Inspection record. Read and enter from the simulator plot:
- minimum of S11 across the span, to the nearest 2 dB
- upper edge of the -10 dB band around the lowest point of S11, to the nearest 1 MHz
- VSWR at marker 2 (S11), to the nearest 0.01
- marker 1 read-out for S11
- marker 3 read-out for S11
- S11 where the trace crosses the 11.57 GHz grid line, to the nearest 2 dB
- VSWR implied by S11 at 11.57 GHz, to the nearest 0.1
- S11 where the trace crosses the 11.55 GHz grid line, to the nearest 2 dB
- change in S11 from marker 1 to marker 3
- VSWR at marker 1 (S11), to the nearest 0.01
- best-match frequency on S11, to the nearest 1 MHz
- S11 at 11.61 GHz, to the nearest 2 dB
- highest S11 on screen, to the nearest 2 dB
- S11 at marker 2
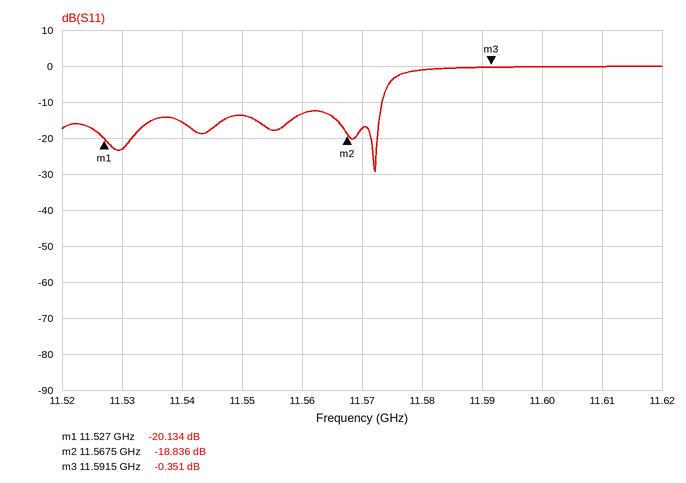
-30 dB
11.573 GHz
1.26
-20.134 dB
-0.351 dB
-18 dB
1.3
-14 dB
19.783 dB
1.22
11.572 GHz
0 dB
0 dB
-18.836 dB
